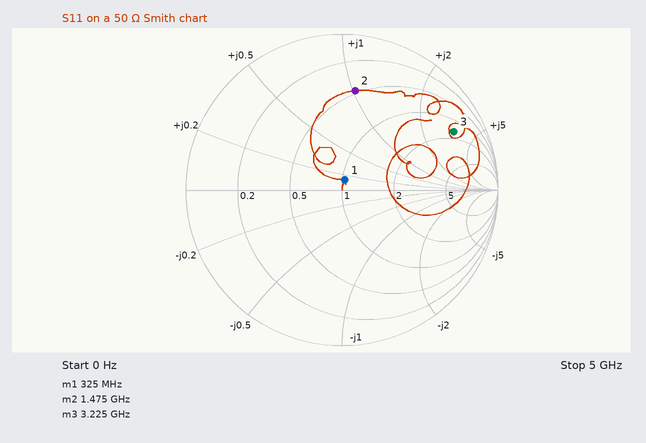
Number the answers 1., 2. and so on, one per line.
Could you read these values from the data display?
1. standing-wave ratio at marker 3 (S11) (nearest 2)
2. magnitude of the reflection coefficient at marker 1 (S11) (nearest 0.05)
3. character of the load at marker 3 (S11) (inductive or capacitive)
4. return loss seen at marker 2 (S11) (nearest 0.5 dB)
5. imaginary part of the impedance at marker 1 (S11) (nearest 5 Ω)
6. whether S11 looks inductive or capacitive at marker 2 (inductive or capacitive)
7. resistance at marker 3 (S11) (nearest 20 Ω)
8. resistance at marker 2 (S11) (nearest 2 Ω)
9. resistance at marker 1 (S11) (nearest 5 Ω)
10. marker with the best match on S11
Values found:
1. 10
2. 0.05
3. inductive
4. 4.0 dB
5. +5 Ω
6. inductive
7. 80 Ω
8. 24 Ω
9. 50 Ω
10. marker 1
